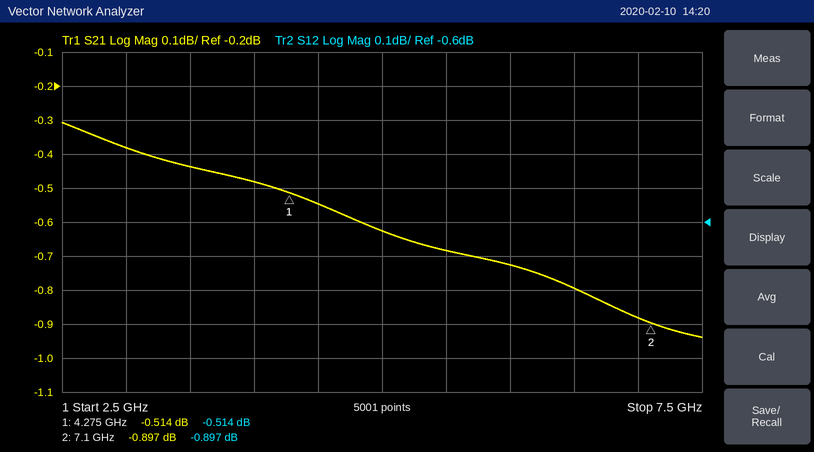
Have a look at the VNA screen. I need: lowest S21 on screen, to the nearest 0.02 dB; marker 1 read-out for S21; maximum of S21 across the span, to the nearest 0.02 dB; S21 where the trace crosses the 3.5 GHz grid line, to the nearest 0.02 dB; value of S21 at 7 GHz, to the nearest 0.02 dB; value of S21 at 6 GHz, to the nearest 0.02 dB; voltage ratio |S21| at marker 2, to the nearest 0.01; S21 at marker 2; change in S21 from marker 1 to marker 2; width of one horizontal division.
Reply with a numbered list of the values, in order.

1. -0.94 dB
2. -0.514 dB
3. -0.30 dB
4. -0.44 dB
5. -0.88 dB
6. -0.72 dB
7. 0.90
8. -0.897 dB
9. -0.383 dB
10. 500 MHz
